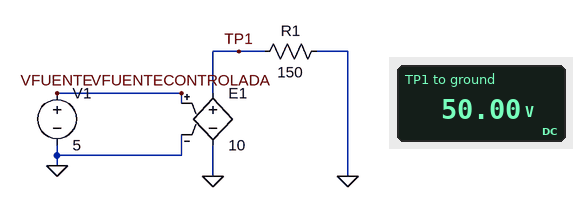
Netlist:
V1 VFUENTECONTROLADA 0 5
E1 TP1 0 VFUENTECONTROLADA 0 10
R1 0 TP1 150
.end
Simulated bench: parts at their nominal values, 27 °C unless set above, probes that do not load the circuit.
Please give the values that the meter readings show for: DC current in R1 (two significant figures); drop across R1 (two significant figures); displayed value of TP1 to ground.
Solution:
330 mA
50 V
50.00 V
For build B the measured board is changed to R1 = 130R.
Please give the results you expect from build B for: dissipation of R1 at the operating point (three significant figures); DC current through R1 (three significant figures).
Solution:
19.2 W
385 mA
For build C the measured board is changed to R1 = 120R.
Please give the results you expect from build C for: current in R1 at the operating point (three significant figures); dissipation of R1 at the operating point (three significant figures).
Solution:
417 mA
20.8 W
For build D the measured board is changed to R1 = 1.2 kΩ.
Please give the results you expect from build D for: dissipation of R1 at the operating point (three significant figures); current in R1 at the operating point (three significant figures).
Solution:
2.08 W
41.7 mA
